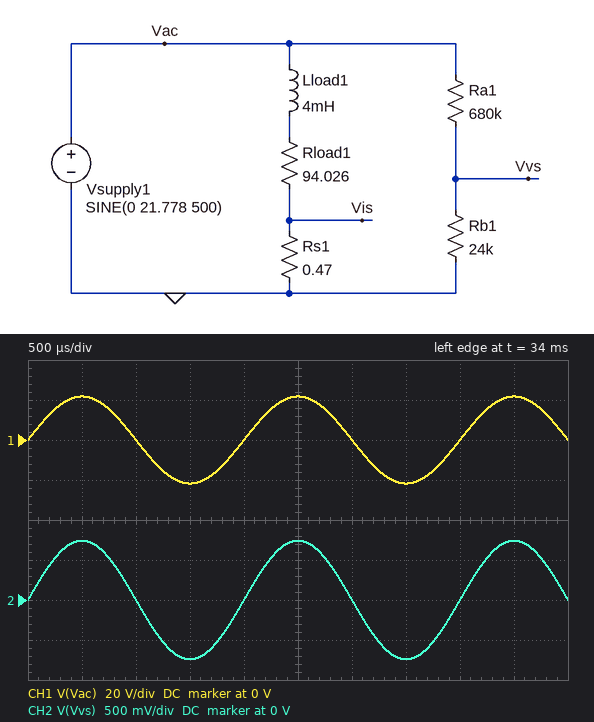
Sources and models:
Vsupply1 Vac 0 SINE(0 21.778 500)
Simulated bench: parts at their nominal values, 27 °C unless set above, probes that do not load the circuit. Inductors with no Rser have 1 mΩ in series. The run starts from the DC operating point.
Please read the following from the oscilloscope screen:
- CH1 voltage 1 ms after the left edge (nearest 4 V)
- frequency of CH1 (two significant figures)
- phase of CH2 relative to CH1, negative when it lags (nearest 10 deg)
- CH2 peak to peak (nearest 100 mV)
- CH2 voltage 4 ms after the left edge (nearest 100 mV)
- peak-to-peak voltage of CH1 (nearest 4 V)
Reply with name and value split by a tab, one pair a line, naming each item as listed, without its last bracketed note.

CH1 voltage 1 ms after the left edge	0 V
frequency of CH1	500 Hz
phase of CH2 relative to CH1, negative when it lags	0 deg
CH2 peak to peak	1.5 V
CH2 voltage 4 ms after the left edge	0 V
peak-to-peak voltage of CH1	44 V
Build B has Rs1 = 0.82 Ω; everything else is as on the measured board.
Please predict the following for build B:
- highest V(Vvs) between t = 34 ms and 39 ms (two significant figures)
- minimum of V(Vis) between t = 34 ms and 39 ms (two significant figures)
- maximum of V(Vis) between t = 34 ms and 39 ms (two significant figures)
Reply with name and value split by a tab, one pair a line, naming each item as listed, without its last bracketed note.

highest V(Vvs) between t = 34 ms and 39 ms	740 mV
minimum of V(Vis) between t = 34 ms and 39 ms	-190 mV
maximum of V(Vis) between t = 34 ms and 39 ms	190 mV
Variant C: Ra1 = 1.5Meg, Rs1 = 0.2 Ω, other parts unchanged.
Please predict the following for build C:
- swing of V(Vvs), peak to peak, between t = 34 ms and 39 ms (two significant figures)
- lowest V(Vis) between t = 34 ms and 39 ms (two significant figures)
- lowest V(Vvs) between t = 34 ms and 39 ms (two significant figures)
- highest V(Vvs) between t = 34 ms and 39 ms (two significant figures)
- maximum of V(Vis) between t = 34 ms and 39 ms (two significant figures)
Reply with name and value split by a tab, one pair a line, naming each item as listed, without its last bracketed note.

swing of V(Vvs), peak to peak, between t = 34 ms and 39 ms	690 mV
lowest V(Vis) between t = 34 ms and 39 ms	-46 mV
lowest V(Vvs) between t = 34 ms and 39 ms	-340 mV
highest V(Vvs) between t = 34 ms and 39 ms	340 mV
maximum of V(Vis) between t = 34 ms and 39 ms	46 mV
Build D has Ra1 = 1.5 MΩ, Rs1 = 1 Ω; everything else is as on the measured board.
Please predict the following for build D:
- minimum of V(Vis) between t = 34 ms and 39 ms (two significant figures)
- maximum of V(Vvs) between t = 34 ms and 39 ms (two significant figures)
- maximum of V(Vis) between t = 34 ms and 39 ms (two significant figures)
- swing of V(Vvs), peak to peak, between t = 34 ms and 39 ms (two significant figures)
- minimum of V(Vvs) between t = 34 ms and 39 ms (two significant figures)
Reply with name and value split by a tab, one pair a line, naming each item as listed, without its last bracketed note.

minimum of V(Vis) between t = 34 ms and 39 ms	-230 mV
maximum of V(Vvs) between t = 34 ms and 39 ms	340 mV
maximum of V(Vis) between t = 34 ms and 39 ms	230 mV
swing of V(Vvs), peak to peak, between t = 34 ms and 39 ms	690 mV
minimum of V(Vvs) between t = 34 ms and 39 ms	-340 mV
